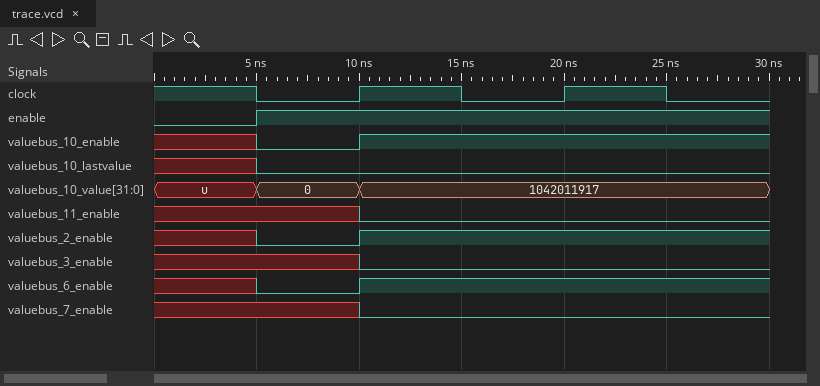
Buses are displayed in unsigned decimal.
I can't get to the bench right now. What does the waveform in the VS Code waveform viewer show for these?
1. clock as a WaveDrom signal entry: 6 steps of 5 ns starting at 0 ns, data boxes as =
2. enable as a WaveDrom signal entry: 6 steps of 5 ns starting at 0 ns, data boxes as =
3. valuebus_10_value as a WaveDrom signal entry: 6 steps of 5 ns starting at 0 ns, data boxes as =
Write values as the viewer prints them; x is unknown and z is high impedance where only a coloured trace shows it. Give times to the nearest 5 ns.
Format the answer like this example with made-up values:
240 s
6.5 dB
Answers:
{name: 'clock', wave: '101010'}
{name: 'enable', wave: '01....'}
{name: 'valuebus_10_value', wave: 'x==...', data: '0 1042011917'}
